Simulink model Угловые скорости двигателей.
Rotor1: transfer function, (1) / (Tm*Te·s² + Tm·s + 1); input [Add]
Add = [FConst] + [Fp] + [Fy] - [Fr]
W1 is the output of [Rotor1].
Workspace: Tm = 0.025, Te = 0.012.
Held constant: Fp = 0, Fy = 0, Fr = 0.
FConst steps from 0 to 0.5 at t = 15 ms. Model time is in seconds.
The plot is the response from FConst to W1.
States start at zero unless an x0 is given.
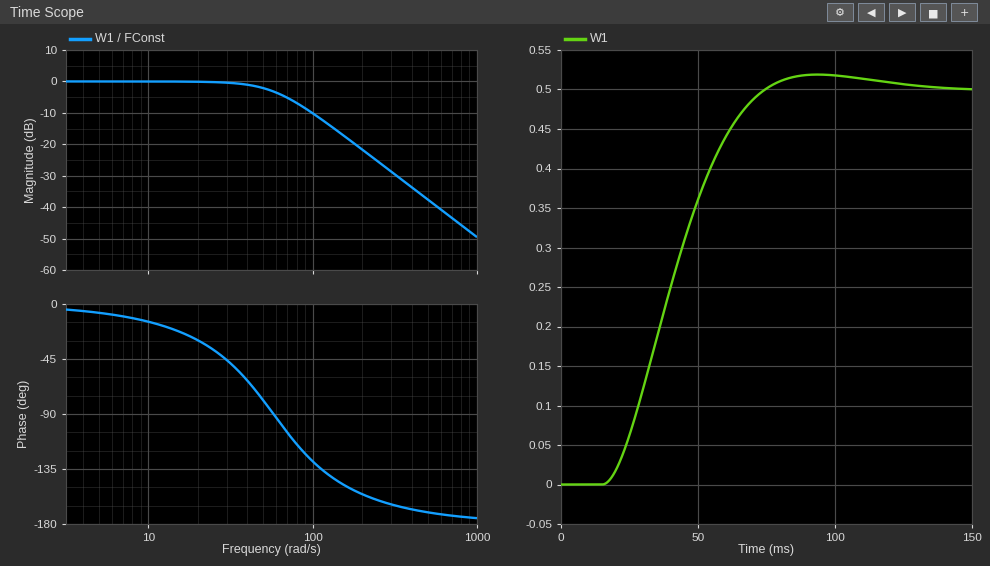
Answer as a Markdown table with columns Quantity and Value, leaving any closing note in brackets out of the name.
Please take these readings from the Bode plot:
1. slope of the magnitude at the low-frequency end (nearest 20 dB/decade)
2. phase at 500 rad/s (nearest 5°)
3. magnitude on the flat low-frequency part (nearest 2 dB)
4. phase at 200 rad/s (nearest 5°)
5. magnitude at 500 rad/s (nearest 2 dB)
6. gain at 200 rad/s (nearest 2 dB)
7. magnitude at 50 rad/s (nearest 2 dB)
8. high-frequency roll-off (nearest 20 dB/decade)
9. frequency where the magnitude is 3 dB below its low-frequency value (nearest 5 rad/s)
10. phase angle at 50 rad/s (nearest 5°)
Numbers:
| Quantity | Value |
|---|---|
| slope of the magnitude at the low-frequency end | 0 dB/decade |
| phase at 500 rad/s | -170° |
| magnitude on the flat low-frequency part | 0 dB |
| phase at 200 rad/s | -155° |
| magnitude at 500 rad/s | -38 dB |
| gain at 200 rad/s | -22 dB |
| magnitude at 50 rad/s | -2 dB |
| high-frequency roll-off | -40 dB/decade |
| frequency where the magnitude is 3 dB below its low-frequency value | 55 rad/s |
| phase angle at 50 rad/s | -80° |
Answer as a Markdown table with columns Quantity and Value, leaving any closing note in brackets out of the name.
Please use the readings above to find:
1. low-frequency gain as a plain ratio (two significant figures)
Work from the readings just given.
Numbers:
| Quantity | Value |
|---|---|
| low-frequency gain as a plain ratio | 1.0 |
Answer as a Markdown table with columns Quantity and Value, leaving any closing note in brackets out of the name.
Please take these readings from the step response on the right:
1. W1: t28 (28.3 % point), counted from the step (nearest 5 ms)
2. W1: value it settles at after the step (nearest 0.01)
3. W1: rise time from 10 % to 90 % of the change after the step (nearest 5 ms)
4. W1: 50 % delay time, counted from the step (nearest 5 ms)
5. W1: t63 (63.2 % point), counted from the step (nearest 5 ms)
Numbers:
| Quantity | Value |
|---|---|
| W1: t28 (28.3 % point), counted from the step | 15 ms |
| W1: value it settles at after the step | 0.50 |
| W1: rise time from 10 % to 90 % of the change after the step | 40 ms |
| W1: 50 % delay time, counted from the step | 25 ms |
| W1: t63 (63.2 % point), counted from the step | 30 ms |
